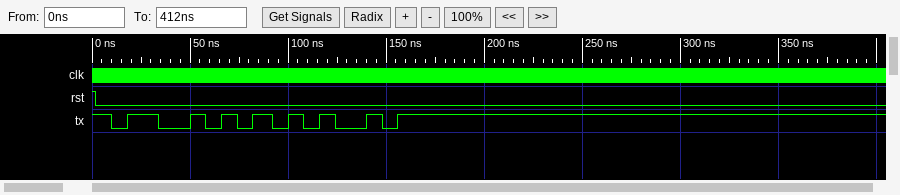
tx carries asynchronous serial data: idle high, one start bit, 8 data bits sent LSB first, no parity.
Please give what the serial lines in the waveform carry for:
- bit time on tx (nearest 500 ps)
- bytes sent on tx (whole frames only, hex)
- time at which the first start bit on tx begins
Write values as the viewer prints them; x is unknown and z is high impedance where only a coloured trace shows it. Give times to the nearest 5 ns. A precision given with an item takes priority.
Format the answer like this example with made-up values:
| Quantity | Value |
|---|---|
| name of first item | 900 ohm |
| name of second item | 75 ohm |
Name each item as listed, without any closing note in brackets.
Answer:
| Quantity | Value |
|---|---|
| bit time on tx | 8000 ps |
| bytes sent on tx | 53, A5 |
| time at which the first start bit on tx begins | 10 ns |
